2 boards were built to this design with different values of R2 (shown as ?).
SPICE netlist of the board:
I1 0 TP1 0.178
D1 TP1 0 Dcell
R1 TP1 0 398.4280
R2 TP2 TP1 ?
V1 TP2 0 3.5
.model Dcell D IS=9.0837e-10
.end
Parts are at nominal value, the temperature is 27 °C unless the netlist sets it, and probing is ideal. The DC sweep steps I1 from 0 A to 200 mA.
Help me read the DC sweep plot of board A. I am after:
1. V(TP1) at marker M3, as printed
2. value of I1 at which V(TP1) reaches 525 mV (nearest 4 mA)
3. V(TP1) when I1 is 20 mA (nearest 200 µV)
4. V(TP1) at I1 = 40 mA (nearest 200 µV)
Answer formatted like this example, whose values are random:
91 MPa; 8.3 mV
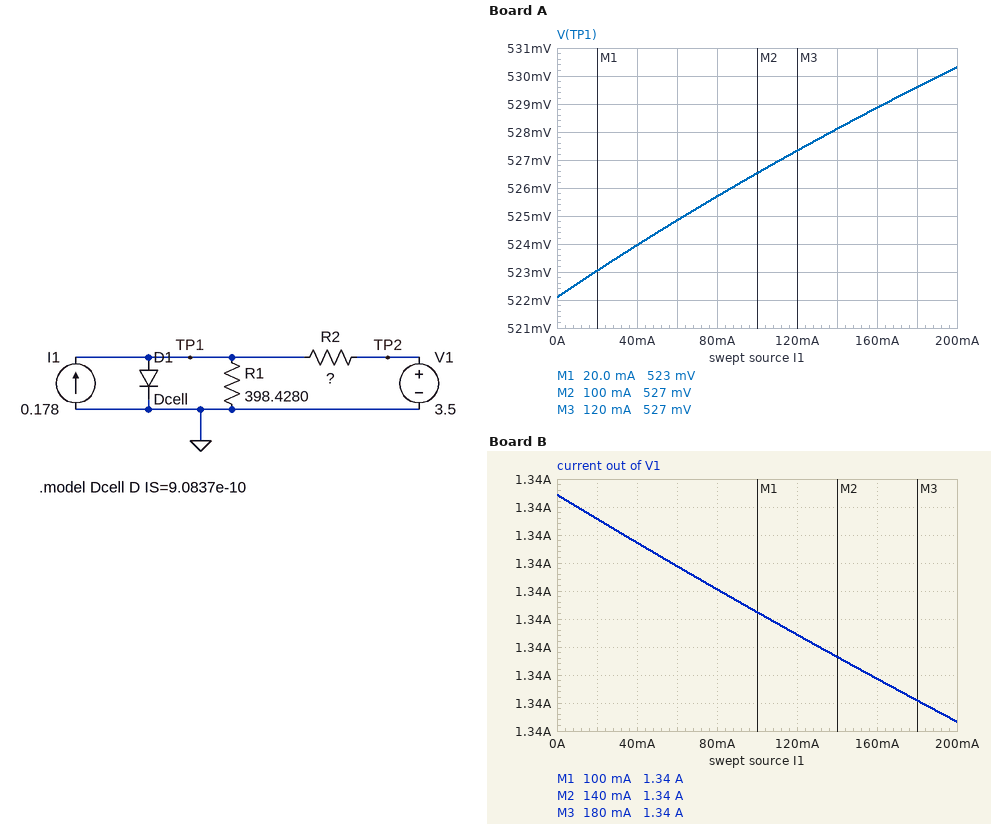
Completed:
527 mV; 64 mA; 523.0 mV; 524.0 mV
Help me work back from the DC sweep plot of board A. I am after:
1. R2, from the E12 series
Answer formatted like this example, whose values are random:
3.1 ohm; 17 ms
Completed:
5.6 Ω
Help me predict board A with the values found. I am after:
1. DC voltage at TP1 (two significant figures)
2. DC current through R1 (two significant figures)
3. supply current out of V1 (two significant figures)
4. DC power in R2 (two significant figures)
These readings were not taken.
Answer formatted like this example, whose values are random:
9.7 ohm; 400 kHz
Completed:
530 mV; 1.3 mA; 530 mA; 1.6 W
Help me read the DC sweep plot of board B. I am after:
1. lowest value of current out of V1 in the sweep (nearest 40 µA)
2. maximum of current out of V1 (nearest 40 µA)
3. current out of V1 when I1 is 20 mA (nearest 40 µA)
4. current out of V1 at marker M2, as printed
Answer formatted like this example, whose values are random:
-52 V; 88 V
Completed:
1.34108 A; 1.34268 A; 1.34252 A; 1.34 A
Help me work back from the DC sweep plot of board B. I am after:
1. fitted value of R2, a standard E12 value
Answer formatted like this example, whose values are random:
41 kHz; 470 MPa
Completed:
2.2 Ω
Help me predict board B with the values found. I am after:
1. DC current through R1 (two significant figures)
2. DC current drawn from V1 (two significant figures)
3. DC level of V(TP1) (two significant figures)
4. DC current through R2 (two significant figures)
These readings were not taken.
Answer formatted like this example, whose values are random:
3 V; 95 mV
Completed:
1.4 mA; 1.3 A; 550 mV; 1.3 A
